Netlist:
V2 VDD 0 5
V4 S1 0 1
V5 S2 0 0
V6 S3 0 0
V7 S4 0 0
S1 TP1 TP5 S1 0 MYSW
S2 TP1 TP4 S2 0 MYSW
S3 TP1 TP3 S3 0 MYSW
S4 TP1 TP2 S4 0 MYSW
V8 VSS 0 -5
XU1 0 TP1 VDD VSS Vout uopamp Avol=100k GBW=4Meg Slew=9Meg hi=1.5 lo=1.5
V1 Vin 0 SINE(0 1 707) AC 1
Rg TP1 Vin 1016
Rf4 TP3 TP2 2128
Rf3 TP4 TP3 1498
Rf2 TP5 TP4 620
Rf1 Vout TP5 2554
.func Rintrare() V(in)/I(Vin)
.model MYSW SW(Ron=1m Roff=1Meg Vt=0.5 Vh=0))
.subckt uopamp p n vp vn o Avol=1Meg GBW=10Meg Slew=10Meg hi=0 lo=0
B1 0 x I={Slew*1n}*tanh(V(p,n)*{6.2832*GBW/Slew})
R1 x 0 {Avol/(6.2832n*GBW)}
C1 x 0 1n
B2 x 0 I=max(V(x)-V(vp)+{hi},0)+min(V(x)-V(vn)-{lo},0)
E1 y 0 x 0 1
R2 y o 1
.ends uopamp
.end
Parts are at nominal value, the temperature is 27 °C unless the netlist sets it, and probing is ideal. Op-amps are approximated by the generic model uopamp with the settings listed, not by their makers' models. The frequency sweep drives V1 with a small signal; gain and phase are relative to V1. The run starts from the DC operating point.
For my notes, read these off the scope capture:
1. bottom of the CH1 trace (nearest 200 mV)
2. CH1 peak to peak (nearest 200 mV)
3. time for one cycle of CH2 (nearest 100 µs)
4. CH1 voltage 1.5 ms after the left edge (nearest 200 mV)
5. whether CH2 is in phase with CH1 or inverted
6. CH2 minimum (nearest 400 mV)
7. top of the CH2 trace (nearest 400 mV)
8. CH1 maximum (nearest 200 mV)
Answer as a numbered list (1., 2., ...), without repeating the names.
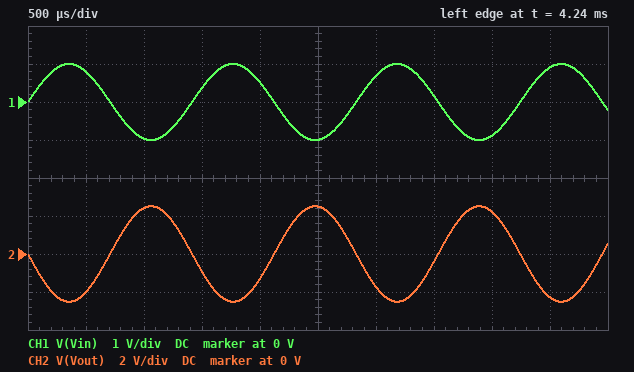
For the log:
1. -1.0 V
2. 2.0 V
3. 1.4 ms
4. 400 mV
5. inverted
6. -2.4 V
7. 2.4 V
8. 1.0 V
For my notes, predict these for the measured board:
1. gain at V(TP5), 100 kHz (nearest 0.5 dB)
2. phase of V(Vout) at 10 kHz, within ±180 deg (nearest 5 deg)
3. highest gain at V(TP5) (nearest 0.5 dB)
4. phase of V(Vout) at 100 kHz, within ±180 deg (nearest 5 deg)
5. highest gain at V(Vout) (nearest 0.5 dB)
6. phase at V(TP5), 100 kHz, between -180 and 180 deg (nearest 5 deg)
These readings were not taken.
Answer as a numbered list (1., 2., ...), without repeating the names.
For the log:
1. 32.0 dB
2. 150 deg
3. 48.0 dB
4. 100 deg
5. 48.0 dB
6. 100 deg
